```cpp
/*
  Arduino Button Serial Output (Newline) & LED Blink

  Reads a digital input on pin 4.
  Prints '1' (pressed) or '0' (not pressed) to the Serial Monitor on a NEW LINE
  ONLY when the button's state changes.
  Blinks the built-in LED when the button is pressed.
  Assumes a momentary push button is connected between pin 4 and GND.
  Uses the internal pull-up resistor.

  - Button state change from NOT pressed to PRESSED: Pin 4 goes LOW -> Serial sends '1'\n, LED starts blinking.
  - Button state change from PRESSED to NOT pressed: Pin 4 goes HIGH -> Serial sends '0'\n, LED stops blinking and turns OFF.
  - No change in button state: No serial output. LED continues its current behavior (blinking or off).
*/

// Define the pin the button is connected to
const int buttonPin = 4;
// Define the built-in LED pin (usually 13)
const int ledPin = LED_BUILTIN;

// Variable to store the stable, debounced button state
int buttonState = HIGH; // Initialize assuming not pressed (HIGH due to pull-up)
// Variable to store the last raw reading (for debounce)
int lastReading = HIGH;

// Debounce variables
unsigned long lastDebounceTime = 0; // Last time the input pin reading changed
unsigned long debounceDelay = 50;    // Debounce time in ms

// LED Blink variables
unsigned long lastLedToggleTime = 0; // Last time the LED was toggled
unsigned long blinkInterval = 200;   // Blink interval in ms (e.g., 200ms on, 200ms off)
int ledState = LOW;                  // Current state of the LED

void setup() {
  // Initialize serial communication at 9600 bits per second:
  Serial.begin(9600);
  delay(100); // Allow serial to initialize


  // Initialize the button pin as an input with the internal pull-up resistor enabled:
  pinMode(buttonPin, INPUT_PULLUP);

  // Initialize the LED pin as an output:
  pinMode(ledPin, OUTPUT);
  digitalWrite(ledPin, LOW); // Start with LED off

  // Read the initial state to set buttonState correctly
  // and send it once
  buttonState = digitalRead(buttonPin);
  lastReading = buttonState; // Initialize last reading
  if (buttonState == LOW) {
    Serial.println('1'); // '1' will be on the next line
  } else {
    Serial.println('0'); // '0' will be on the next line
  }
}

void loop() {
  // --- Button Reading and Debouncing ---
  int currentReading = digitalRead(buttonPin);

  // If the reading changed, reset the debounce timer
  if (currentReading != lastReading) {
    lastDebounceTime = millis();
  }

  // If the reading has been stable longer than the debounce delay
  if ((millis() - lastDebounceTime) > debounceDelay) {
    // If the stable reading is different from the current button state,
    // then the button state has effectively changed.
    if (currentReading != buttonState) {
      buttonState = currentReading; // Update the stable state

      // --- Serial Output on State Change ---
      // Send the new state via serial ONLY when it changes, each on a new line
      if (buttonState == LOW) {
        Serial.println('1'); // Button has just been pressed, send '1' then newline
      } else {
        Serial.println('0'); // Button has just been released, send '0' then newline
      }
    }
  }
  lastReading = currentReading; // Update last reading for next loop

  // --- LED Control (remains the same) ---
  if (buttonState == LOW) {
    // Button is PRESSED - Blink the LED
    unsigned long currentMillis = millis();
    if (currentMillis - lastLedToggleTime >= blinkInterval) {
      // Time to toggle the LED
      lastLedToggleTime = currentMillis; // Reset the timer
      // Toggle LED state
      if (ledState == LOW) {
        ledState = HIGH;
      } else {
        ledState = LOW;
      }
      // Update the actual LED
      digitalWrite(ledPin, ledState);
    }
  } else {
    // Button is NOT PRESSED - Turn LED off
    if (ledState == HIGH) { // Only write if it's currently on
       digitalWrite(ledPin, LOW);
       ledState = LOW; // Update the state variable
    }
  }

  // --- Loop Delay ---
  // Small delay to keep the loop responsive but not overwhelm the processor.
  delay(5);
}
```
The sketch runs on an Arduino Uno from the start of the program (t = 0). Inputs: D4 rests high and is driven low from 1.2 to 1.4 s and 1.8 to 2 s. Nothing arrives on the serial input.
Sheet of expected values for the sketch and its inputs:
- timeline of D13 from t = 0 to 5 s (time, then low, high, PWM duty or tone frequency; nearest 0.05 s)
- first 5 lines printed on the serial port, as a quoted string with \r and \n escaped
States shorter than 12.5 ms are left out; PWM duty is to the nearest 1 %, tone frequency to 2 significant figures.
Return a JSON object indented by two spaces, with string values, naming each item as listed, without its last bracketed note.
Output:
{
  "timeline of D13 from t = 0 to 5 s": "0.1 s low; 1.25 s high; 1.45 s low; 1.85 s high; 2.05 s low",
  "first 5 lines printed on the serial port, as a quoted string with \\r and \\n escaped": "\"0\\r\\n1\\r\\n0\\r\\n1\\r\\n0\\r\\n\""
}
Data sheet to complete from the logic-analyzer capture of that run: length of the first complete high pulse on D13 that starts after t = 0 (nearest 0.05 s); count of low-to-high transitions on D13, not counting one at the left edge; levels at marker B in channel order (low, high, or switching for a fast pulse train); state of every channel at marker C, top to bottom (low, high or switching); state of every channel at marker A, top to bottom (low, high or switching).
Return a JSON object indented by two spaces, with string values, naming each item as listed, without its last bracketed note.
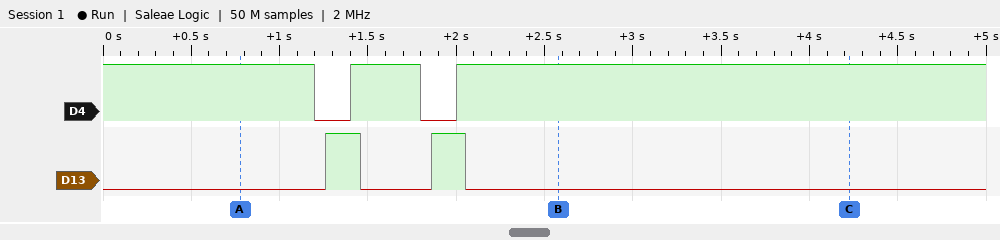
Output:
{
  "length of the first complete high pulse on D13 that starts after t = 0": "0.20 s",
  "count of low-to-high transitions on D13, not counting one at the left edge": "2",
  "levels at marker B in channel order": "D4 high, D13 low",
  "state of every channel at marker C, top to bottom": "D4 high, D13 low",
  "state of every channel at marker A, top to bottom": "D4 high, D13 low"
}
